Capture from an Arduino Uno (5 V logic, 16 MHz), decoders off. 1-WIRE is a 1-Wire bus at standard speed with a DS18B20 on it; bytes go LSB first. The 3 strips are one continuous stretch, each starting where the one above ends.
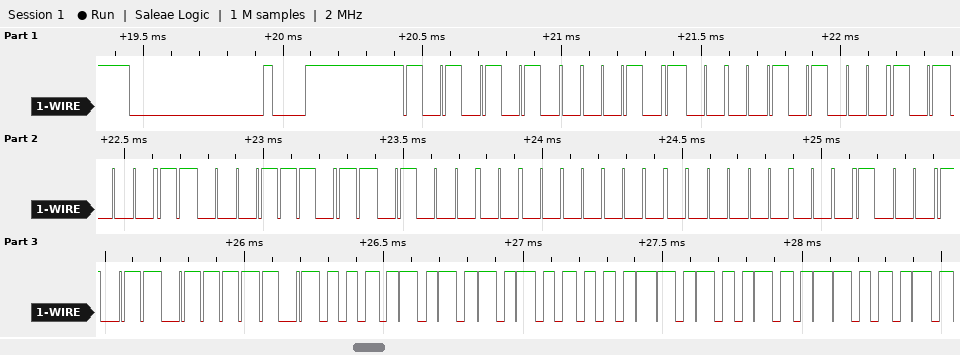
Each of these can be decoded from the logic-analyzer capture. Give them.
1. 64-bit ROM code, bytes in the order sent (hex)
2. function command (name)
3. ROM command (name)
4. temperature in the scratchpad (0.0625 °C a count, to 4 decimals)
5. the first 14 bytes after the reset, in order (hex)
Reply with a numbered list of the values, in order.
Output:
1. 28 14 C5 B8 05 00 00 D1
2. Read Scratchpad
3. Match ROM
4. 85.0000 °C
5. 55 28 14 C5 B8 05 00 00 D1 BE 50 05 4B 46
